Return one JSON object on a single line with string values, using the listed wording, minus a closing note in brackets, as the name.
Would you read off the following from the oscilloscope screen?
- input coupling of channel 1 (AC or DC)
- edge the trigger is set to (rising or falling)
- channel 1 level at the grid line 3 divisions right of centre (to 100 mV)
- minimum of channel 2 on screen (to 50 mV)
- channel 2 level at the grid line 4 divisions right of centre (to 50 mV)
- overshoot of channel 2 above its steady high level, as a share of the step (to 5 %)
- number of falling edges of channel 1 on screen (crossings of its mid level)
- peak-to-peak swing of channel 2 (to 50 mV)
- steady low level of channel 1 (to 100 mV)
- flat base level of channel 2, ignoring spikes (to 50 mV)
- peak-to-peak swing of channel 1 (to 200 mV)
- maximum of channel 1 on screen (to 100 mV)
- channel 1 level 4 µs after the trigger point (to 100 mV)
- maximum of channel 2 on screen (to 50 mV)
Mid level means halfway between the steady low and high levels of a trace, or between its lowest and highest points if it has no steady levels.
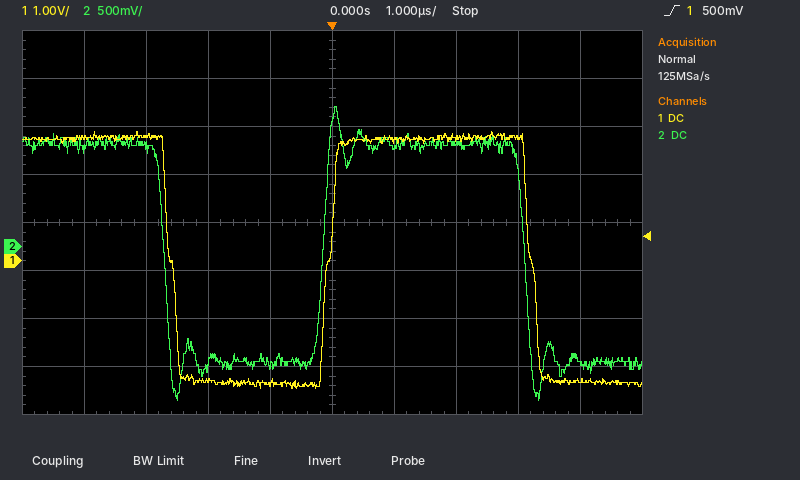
{"input coupling of channel 1": "DC", "edge the trigger is set to": "rising", "channel 1 level at the grid line 3 divisions right of centre": "2.6 V", "minimum of channel 2 on screen": "-1.60 V", "channel 2 level at the grid line 4 divisions right of centre": "-1.20 V", "overshoot of channel 2 above its steady high level, as a share of the step": "15 %", "number of falling edges of channel 1 on screen": "2", "peak-to-peak swing of channel 2": "3.05 V", "steady low level of channel 1": "-2.5 V", "flat base level of channel 2, ignoring spikes": "-1.20 V", "peak-to-peak swing of channel 1": "5.4 V", "maximum of channel 1 on screen": "2.7 V", "channel 1 level 4 µs after the trigger point": "-2.5 V", "maximum of channel 2 on screen": "1.45 V"}
